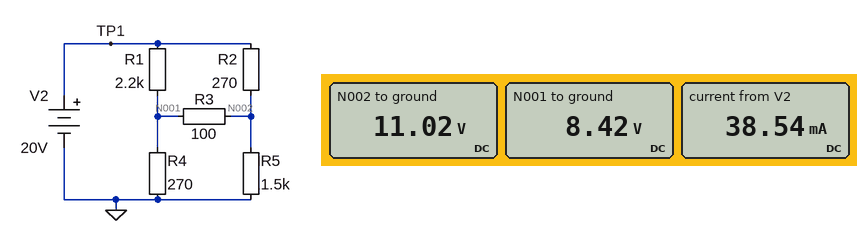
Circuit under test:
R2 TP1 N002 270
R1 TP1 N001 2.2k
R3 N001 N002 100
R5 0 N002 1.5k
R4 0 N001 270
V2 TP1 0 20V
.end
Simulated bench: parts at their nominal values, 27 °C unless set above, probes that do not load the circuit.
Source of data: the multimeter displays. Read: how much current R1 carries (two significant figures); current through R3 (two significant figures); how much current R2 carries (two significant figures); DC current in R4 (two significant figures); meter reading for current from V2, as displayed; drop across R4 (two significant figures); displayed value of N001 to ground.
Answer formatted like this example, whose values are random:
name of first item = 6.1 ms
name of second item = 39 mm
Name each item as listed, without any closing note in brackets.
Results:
how much current R1 carries = 5.3 mA
current through R3 = 26 mA
how much current R2 carries = 33 mA
DC current in R4 = 31 mA
meter reading for current from V2, as displayed = 38.54 mA
drop across R4 = 8.4 V
displayed value of N001 to ground = 8.42 V
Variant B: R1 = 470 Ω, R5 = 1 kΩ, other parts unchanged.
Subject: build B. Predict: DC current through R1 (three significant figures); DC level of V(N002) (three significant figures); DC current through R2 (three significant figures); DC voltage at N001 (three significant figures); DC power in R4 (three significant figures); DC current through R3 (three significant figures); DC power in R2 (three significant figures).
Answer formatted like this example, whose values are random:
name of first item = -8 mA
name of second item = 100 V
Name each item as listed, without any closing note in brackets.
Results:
DC current through R1 = 20.7 mA
DC level of V(N002) = 12.0 V
DC current through R2 = 29.5 mA
DC voltage at N001 = 10.3 V
DC power in R4 = 392 mW
DC current through R3 = 17.5 mA
DC power in R2 = 235 mW
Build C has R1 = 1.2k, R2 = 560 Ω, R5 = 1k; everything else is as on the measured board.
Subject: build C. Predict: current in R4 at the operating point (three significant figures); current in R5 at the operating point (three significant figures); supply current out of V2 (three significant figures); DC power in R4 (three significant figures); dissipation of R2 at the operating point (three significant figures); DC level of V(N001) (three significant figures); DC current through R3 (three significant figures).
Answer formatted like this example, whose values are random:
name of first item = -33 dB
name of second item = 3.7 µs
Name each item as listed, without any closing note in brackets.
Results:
current in R4 at the operating point = 24.6 mA
current in R5 at the operating point = 7.99 mA
supply current out of V2 = 32.6 mA
DC power in R4 = 163 mW
dissipation of R2 at the operating point = 258 mW
DC level of V(N001) = 6.64 V
DC current through R3 = 13.5 mA
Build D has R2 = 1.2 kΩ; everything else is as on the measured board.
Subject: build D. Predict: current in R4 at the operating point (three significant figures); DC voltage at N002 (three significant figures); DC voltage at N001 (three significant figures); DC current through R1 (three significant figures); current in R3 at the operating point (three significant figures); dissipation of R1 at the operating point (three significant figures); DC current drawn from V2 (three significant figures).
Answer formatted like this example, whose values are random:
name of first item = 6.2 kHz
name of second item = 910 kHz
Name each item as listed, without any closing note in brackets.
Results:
current in R4 at the operating point = 16.0 mA
DC voltage at N002 = 5.20 V
DC voltage at N001 = 4.32 V
DC current through R1 = 7.13 mA
current in R3 at the operating point = 8.86 mA
dissipation of R1 at the operating point = 112 mW
DC current drawn from V2 = 19.5 mA
